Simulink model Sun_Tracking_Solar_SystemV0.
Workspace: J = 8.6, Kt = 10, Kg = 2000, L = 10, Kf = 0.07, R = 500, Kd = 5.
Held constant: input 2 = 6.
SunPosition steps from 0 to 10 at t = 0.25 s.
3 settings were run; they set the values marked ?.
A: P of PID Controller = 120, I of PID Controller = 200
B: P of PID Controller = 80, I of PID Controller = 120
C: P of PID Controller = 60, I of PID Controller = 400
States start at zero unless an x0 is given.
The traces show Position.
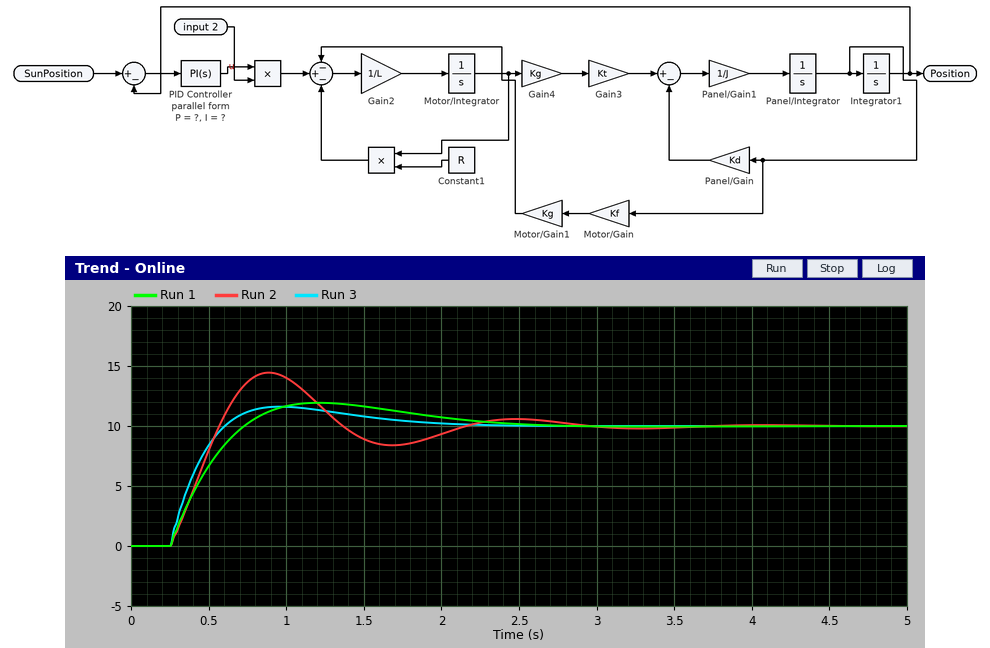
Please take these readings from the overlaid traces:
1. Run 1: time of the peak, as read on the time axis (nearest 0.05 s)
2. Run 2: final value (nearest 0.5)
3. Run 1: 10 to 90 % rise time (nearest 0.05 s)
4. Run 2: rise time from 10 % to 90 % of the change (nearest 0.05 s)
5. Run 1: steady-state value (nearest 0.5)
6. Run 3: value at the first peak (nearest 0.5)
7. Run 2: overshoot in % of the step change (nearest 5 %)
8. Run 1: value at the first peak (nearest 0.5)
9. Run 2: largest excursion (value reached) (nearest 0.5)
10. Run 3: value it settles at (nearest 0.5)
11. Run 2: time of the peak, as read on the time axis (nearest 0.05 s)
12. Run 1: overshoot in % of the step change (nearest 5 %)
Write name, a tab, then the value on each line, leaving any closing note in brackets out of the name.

Run 1: time of the peak, as read on the time axis	1.20 s
Run 2: final value	10.0
Run 1: 10 to 90 % rise time	0.35 s
Run 2: rise time from 10 % to 90 % of the change	0.25 s
Run 1: steady-state value	10.0
Run 3: value at the first peak	11.5
Run 2: overshoot in % of the step change	45 %
Run 1: value at the first peak	12.0
Run 2: largest excursion (value reached)	14.5
Run 3: value it settles at	10.0
Run 2: time of the peak, as read on the time axis	0.90 s
Run 1: overshoot in % of the step change	20 %
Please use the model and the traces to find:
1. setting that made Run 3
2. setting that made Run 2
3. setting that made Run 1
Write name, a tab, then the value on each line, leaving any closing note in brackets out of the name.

setting that made Run 3	A
setting that made Run 2	C
setting that made Run 1	B
